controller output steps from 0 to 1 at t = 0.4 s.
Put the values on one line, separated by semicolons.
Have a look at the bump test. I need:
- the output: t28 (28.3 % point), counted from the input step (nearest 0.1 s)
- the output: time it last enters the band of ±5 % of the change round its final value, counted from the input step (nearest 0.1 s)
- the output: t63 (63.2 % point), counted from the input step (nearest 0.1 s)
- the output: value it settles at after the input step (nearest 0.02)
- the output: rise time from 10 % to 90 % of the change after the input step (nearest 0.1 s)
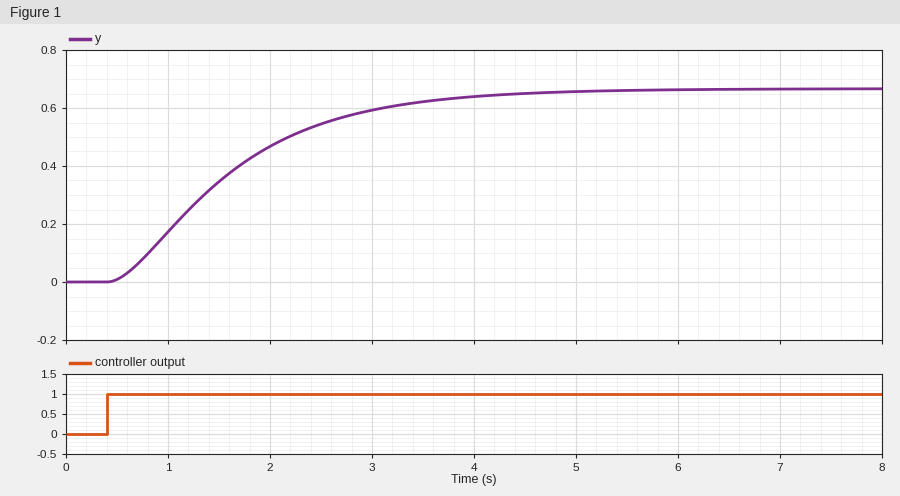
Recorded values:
0.6 s; 3.4 s; 1.4 s; 0.66; 2.4 s
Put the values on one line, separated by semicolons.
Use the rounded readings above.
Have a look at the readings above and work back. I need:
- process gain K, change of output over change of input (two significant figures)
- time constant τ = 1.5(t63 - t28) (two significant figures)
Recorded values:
0.66; 1.2 s
